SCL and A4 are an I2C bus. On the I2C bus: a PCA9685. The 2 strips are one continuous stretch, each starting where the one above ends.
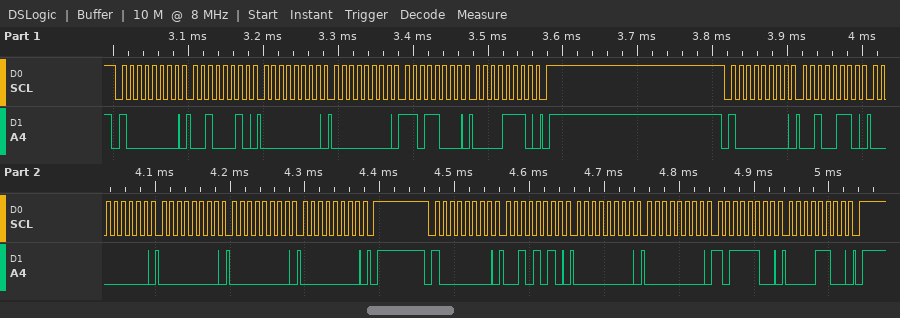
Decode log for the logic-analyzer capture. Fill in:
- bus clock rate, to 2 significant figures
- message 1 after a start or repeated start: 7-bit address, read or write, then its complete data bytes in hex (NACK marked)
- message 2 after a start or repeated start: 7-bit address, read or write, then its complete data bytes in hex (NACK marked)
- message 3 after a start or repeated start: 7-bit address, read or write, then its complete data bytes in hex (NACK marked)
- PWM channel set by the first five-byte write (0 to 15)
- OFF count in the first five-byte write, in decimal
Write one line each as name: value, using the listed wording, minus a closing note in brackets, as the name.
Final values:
bus clock rate, to 2 significant figures: 100 kHz
message 1 after a start or repeated start: 7-bit address, read or write, then its complete data bytes in hex: 0x40 write: 22 00 00 D8 0E
message 2 after a start or repeated start: 7-bit address, read or write, then its complete data bytes in hex: 0x40 write: 26 00 00 00 00
message 3 after a start or repeated start: 7-bit address, read or write, then its complete data bytes in hex: 0x40 write: 2A 00 00 BC 0C
PWM channel set by the first five-byte write: 7
OFF count in the first five-byte write, in decimal: 3800
